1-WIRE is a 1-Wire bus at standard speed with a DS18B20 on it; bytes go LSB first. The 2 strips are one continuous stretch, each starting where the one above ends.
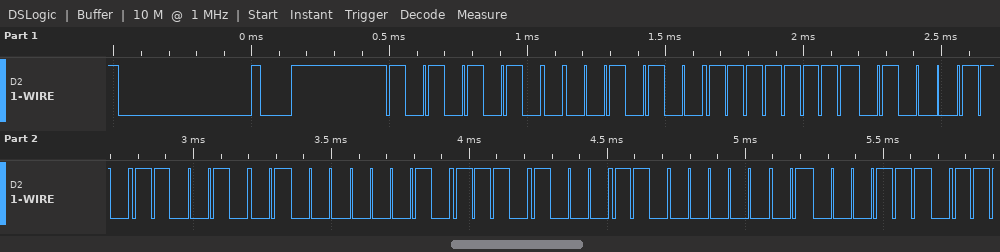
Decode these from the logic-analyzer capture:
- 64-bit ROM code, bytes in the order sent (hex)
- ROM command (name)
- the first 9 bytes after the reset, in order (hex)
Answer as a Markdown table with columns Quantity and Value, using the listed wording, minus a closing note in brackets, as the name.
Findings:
| Quantity | Value |
|---|---|
| 64-bit ROM code, bytes in the order sent | 28 FF 62 93 40 17 03 E2 |
| ROM command | Match ROM |
| the first 9 bytes after the reset, in order | 55 28 FF 62 93 40 17 03 E2 |
